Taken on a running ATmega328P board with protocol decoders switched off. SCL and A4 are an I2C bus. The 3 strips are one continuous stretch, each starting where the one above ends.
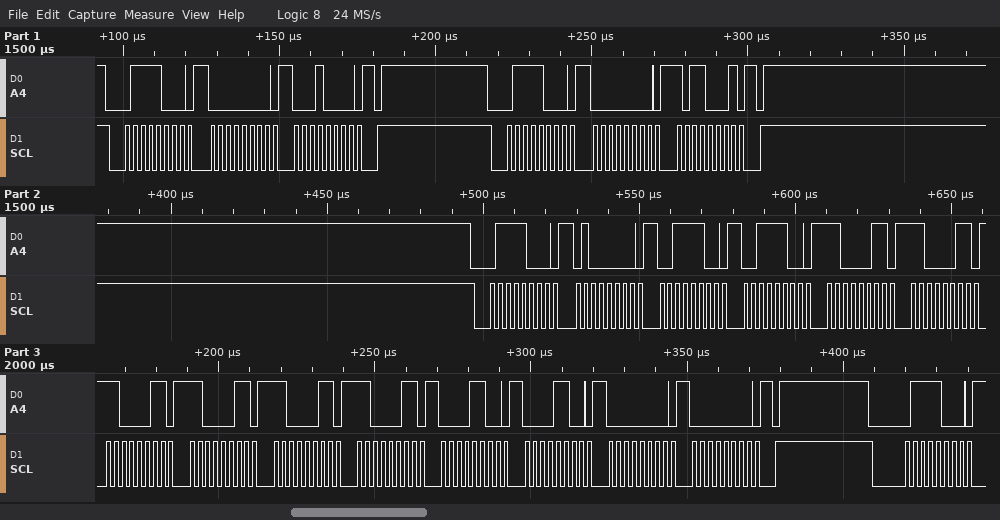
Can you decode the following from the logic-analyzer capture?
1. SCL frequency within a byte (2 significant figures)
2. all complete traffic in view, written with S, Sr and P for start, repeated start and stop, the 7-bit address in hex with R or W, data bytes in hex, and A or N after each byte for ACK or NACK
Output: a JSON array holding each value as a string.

["400 kHz", "S 3CW A 00 A 10 A P S 3CW A 00 A B1 A P S 3CW A 40 A 3C A 3C A C3 A C3 A C3 A C3 A C3 A C3 A 0C A 0C A 00 A 00 A P S 3CW A"]
